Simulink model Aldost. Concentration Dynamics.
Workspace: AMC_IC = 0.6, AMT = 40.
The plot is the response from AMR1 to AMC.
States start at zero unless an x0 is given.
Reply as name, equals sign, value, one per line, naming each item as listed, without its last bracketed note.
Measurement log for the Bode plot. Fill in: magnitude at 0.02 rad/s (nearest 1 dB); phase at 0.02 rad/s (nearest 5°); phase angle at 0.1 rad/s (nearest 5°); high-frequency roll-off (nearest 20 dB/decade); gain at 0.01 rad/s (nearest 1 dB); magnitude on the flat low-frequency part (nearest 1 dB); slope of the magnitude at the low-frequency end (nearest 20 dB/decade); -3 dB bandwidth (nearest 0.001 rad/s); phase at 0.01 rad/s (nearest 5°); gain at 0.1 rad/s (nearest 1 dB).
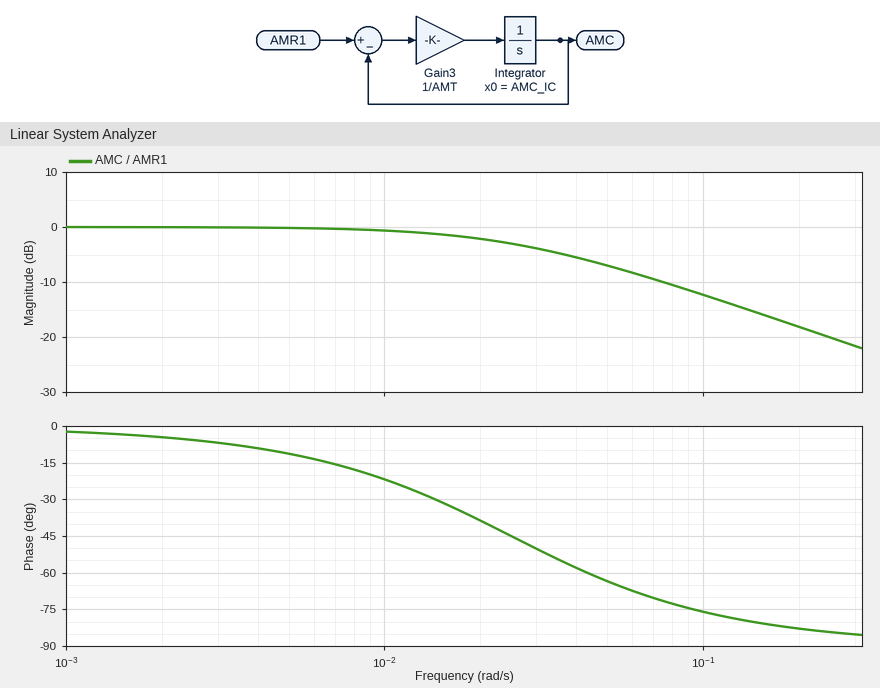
magnitude at 0.02 rad/s = -2 dB
phase at 0.02 rad/s = -40°
phase angle at 0.1 rad/s = -75°
high-frequency roll-off = -20 dB/decade
gain at 0.01 rad/s = -1 dB
magnitude on the flat low-frequency part = 0 dB
slope of the magnitude at the low-frequency end = 0 dB/decade
-3 dB bandwidth = 0.025 rad/s
phase at 0.01 rad/s = -20°
gain at 0.1 rad/s = -12 dB
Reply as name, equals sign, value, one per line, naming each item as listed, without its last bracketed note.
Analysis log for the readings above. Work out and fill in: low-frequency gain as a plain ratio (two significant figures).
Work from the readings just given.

low-frequency gain as a plain ratio = 1.0
